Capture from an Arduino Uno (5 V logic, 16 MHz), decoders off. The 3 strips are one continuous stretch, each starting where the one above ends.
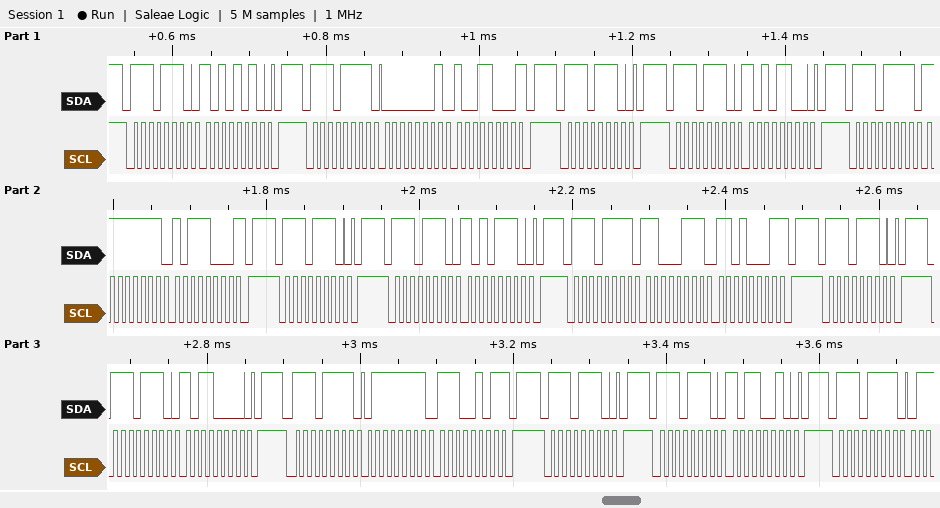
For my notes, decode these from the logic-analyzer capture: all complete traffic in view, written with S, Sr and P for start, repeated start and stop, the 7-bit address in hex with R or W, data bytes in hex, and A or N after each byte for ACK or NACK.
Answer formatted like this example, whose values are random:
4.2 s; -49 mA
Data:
S 77W A AA A P S 77R A 01 A 98 N P S 77W A P S 77W A AC A P S 77R A FF A B8 N P S 77W A P S 77W A AE A P S 77R A C7 A D1 N P S 77W A P S 77W A B0 A P S 77R A 7F A E5 N P S 77W A P S 77W A B2 A P S 77R A
